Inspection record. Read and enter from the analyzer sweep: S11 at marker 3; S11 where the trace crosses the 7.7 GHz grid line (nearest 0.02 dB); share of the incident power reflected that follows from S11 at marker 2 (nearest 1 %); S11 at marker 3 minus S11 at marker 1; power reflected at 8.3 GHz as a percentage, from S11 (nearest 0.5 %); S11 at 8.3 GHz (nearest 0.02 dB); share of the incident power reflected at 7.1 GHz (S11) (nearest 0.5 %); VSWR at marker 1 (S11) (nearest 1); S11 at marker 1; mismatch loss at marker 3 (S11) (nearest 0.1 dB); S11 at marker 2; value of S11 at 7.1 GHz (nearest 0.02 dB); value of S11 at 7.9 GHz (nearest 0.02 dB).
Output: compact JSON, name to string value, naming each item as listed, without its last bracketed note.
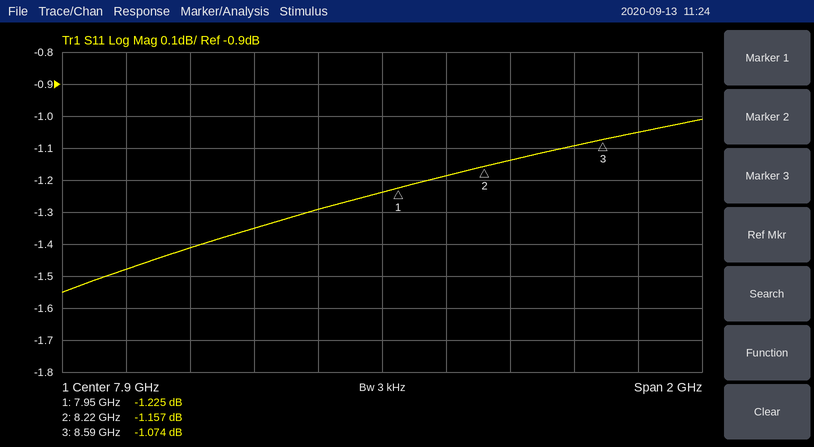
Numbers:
{"S11 at marker 3": "-1.074 dB", "S11 where the trace crosses the 7.7 GHz grid line": "-1.30 dB", "share of the incident power reflected that follows from S11 at marker 2": "77 %", "S11 at marker 3 minus S11 at marker 1": "0.151 dB", "power reflected at 8.3 GHz as a percentage, from S11": "77.0 %", "S11 at 8.3 GHz": "-1.14 dB", "share of the incident power reflected at 7.1 GHz (S11)": "71.0 %", "VSWR at marker 1 (S11)": "14", "S11 at marker 1": "-1.225 dB", "mismatch loss at marker 3 (S11)": "6.6 dB", "S11 at marker 2": "-1.157 dB", "value of S11 at 7.1 GHz": "-1.48 dB", "value of S11 at 7.9 GHz": "-1.24 dB"}
